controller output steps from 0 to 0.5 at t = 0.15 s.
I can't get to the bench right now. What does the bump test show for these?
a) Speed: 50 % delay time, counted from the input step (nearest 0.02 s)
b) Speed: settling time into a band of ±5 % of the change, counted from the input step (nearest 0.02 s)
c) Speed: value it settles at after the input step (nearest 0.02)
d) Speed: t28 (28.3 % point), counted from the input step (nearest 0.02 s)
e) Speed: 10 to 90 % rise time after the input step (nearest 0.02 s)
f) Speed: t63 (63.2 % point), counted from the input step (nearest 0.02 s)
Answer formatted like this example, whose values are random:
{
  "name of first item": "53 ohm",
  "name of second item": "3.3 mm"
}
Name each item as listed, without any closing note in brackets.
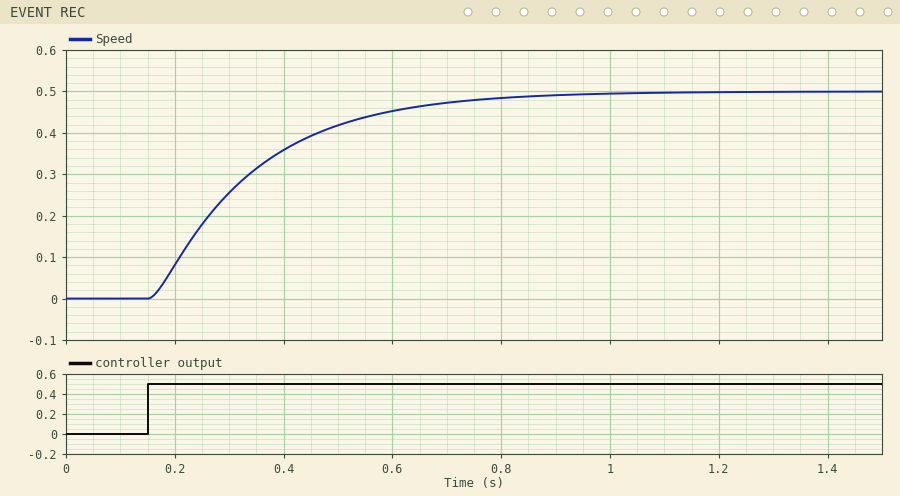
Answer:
{
  "Speed: 50 % delay time, counted from the input step": "0.14 s",
  "Speed: settling time into a band of ±5 % of the change, counted from the input step": "0.56 s",
  "Speed: value it settles at after the input step": "0.50",
  "Speed: t28 (28.3 % point), counted from the input step": "0.08 s",
  "Speed: 10 to 90 % rise time after the input step": "0.40 s",
  "Speed: t63 (63.2 % point), counted from the input step": "0.20 s"
}
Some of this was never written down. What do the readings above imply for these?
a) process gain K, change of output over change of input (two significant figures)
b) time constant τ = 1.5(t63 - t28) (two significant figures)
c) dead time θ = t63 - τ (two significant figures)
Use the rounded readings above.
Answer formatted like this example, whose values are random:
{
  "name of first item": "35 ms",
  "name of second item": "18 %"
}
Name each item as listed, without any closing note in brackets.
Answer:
{
  "process gain K, change of output over change of input": "1.0",
  "time constant τ = 1.5(t63 - t28)": "0.18 s",
  "dead time θ = t63 - τ": "0.020 s"
}
